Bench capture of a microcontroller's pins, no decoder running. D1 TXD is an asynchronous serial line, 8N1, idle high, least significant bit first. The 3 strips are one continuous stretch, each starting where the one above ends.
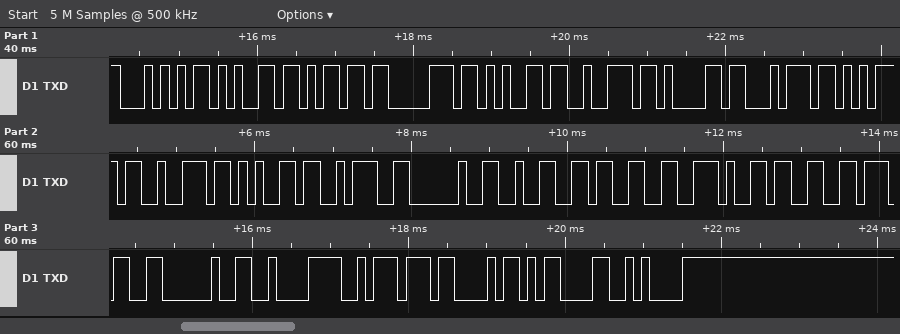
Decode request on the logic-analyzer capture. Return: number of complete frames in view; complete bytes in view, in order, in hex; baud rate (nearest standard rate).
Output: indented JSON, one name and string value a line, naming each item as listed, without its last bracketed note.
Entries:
{
  "number of complete frames in view": "24",
  "complete bytes in view, in order, in hex": "54 65 6D 70 65 72 61 74 75 72 65 3A 20 32 33 2E 33 37 20 C2 BA 43 0D 0A",
  "baud rate": "9600 baud"
}
